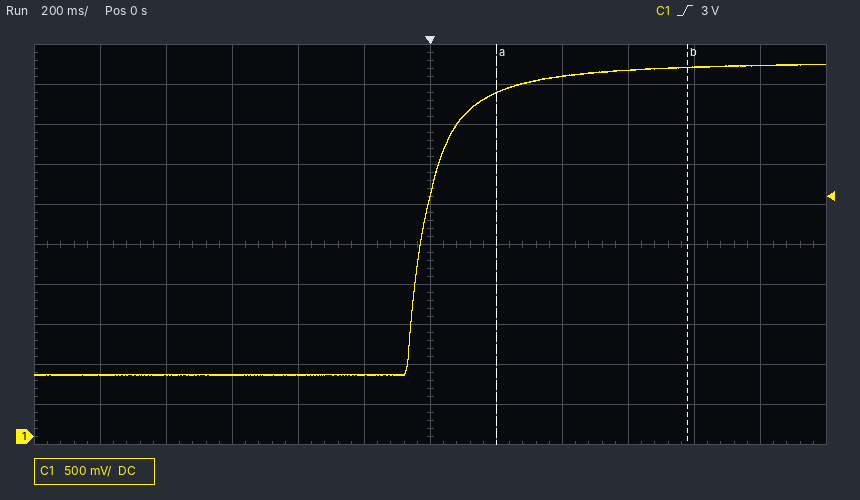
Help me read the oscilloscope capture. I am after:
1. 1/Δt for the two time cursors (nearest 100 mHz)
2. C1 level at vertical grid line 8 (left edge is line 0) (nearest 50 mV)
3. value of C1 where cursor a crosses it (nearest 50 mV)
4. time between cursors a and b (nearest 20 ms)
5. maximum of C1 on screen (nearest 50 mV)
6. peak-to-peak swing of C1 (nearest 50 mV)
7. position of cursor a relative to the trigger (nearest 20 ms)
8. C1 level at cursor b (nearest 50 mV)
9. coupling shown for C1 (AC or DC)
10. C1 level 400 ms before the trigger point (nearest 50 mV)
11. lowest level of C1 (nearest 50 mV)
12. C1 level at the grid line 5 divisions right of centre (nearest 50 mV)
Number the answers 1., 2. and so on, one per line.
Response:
1. 1.7 Hz
2. 4.50 V
3. 4.30 V
4. 580 ms
5. 4.65 V
6. 3.90 V
7. +200 ms
8. 4.60 V
9. DC
10. 750 mV
11. 750 mV
12. 4.65 V
